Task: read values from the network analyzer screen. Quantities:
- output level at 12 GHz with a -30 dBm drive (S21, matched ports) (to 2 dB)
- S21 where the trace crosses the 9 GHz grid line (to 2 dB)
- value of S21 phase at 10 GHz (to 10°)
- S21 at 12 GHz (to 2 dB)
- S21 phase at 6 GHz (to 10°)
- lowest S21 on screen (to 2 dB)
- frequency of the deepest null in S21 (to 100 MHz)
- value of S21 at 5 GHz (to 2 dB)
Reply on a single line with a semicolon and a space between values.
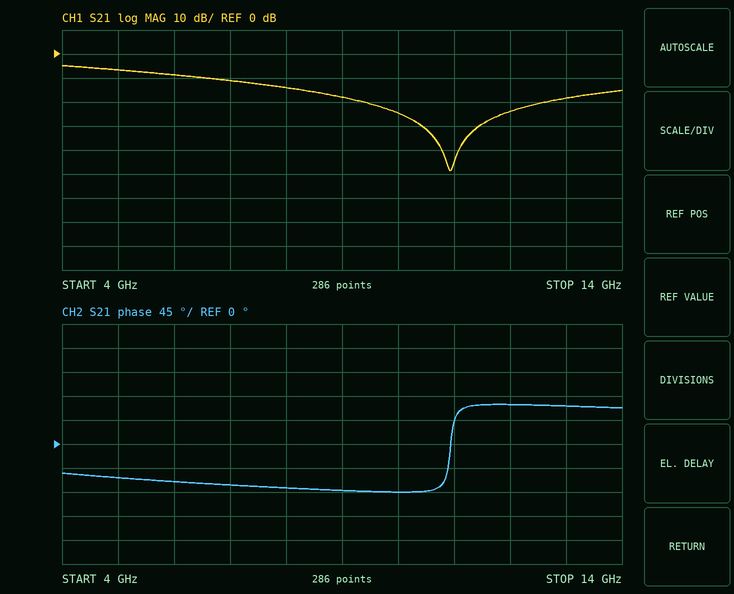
-54 dBm; -18 dB; -90°; -24 dB; -70°; -48 dB; 10.9 GHz; -6 dB
